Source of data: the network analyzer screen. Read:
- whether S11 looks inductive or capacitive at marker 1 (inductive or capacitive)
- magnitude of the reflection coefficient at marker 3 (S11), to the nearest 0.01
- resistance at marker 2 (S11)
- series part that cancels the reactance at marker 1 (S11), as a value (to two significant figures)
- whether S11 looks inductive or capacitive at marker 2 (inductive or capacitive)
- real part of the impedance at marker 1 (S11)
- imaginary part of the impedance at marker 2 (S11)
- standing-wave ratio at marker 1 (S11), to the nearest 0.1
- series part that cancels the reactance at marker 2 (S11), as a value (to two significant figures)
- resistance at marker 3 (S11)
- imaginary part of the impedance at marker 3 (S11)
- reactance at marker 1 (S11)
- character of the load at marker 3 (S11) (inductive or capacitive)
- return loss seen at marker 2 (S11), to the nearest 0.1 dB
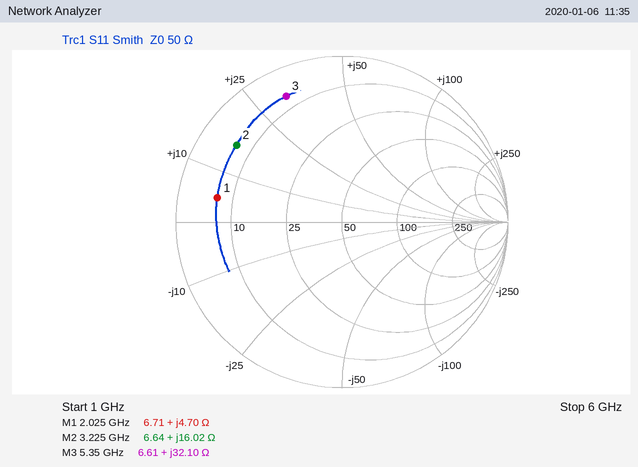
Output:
inductive
0.83
6.64 Ω
17 pF
inductive
6.71 Ω
+16.02 Ω
7.5
3.1 pF
6.61 Ω
+32.10 Ω
+4.70 Ω
inductive
2.1 dB
